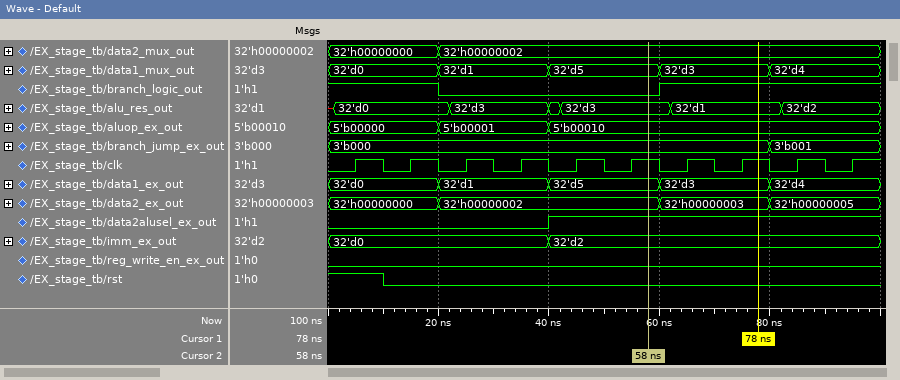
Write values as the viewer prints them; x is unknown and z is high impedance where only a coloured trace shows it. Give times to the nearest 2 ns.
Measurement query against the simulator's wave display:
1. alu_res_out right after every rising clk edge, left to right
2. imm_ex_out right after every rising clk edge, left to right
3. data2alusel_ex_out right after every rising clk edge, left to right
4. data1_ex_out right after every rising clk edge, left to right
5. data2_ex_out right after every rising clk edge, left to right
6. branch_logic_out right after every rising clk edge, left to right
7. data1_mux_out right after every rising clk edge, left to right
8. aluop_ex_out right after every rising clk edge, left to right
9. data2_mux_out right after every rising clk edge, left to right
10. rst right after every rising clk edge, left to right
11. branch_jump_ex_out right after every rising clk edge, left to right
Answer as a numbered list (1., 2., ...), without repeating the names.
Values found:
1. 32'd0, 32'd0, 32'd3, 32'd3, 32'd3, 32'd3, 32'd1, 32'd1, 32'd2, 32'd2
2. 32'd0, 32'd0, 32'd0, 32'd0, 32'd2, 32'd2, 32'd2, 32'd2, 32'd2, 32'd2
3. 0 0 0 0 1 1 1 1 1 1
4. 32'd0, 32'd0, 32'd1, 32'd1, 32'd5, 32'd5, 32'd3, 32'd3, 32'd4, 32'd4
5. 32'h00000000, 32'h00000000, 32'h00000002, 32'h00000002, 32'h00000002, 32'h00000002, 32'h00000003, 32'h00000003, 32'h00000005, 32'h00000005
6. 1 1 0 0 0 0 1 1 1 1
7. 32'd0, 32'd0, 32'd1, 32'd1, 32'd5, 32'd5, 32'd3, 32'd3, 32'd4, 32'd4
8. 5'b00000, 5'b00000, 5'b00001, 5'b00001, 5'b00010, 5'b00010, 5'b00010, 5'b00010, 5'b00010, 5'b00010
9. 32'h00000000, 32'h00000000, 32'h00000002, 32'h00000002, 32'h00000002, 32'h00000002, 32'h00000002, 32'h00000002, 32'h00000002, 32'h00000002
10. 1 0 0 0 0 0 0 0 0 0
11. 3'b000, 3'b000, 3'b000, 3'b000, 3'b000, 3'b000, 3'b000, 3'b000, 3'b001, 3'b001
